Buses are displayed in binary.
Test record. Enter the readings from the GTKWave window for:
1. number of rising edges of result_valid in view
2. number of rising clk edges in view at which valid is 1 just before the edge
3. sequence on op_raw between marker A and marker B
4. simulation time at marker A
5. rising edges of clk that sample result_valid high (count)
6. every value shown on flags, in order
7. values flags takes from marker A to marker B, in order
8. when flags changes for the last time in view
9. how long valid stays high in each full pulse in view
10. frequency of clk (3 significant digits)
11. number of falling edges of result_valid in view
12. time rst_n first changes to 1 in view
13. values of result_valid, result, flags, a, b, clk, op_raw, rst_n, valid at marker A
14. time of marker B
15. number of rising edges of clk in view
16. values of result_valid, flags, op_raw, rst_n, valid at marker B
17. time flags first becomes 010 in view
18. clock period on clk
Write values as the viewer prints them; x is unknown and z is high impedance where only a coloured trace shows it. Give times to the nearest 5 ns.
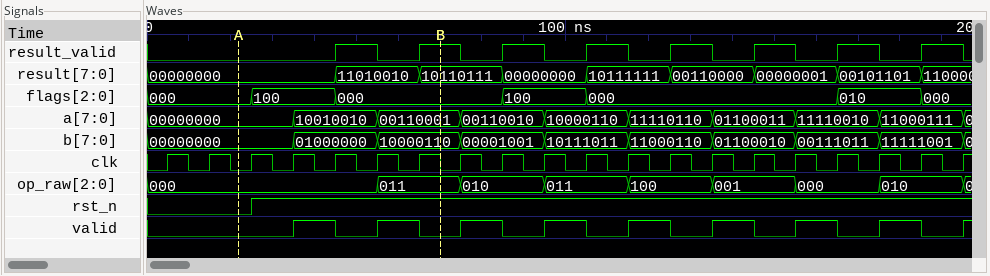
8
8
000, 011
20 ns
8
000, 100, 000, 100, 000, 010, 000
000, 100, 000
185 ns
10 ns, 10 ns, 10 ns, 10 ns, 10 ns, 10 ns, 10 ns, 10 ns
100 MHz
8
25 ns
result_valid=0, result=00000000, flags=000, a=00000000, b=00000000, clk=0, op_raw=000, rst_n=0, valid=0
70 ns
20
result_valid=1, flags=000, op_raw=011, rst_n=1, valid=0
165 ns
10 ns
